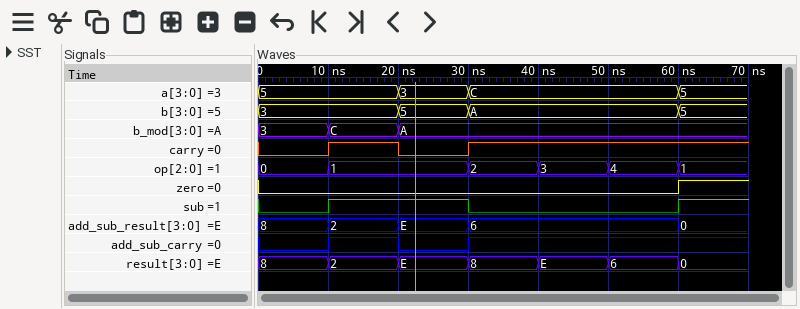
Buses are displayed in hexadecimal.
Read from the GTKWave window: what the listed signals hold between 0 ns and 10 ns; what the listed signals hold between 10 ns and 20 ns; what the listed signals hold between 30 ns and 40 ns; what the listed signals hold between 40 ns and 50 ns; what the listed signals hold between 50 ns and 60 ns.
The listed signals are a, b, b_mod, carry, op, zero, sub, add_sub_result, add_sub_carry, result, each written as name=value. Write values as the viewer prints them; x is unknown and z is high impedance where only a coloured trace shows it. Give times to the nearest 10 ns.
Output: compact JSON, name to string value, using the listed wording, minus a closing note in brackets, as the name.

{"what the listed signals hold between 0 ns and 10 ns": "a=5, b=3, b_mod=3, carry=0, op=0, zero=0, sub=0, add_sub_result=8, add_sub_carry=0, result=8", "what the listed signals hold between 10 ns and 20 ns": "a=5, b=3, b_mod=C, carry=1, op=1, zero=0, sub=1, add_sub_result=2, add_sub_carry=1, result=2", "what the listed signals hold between 30 ns and 40 ns": "a=C, b=A, b_mod=A, carry=1, op=2, zero=0, sub=0, add_sub_result=6, add_sub_carry=1, result=8", "what the listed signals hold between 40 ns and 50 ns": "a=C, b=A, b_mod=A, carry=1, op=3, zero=0, sub=0, add_sub_result=6, add_sub_carry=1, result=E", "what the listed signals hold between 50 ns and 60 ns": "a=C, b=A, b_mod=A, carry=1, op=4, zero=0, sub=0, add_sub_result=6, add_sub_carry=1, result=6"}
